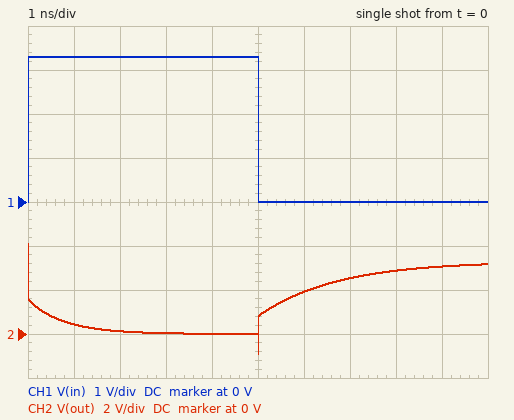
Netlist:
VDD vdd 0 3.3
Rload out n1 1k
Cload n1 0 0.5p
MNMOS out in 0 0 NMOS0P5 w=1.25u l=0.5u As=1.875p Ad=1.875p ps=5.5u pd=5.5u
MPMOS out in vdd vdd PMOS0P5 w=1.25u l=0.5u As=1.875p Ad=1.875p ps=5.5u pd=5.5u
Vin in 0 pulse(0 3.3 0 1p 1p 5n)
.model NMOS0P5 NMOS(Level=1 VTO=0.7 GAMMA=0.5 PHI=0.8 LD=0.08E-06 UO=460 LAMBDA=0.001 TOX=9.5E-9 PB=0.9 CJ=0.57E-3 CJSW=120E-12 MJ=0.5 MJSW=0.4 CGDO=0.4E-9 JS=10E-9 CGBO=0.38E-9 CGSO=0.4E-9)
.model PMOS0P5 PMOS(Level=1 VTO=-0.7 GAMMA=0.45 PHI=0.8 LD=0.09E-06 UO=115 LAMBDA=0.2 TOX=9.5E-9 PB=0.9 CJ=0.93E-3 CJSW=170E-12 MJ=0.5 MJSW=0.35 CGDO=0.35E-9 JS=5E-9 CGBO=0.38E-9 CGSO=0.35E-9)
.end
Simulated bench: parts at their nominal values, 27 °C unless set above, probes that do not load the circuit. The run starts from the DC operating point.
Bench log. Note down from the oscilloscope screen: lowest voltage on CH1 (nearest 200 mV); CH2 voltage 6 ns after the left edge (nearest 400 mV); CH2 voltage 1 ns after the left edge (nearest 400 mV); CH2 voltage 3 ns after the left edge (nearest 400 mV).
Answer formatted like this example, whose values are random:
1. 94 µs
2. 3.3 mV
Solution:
1. 0 V
2. 2.0 V
3. 400 mV
4. 0 V
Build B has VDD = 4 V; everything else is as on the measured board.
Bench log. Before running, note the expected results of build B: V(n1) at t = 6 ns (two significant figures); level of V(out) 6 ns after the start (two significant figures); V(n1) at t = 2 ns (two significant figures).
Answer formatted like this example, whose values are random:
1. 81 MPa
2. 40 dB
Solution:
1. 2.0 V
2. 2.7 V
3. 400 mV
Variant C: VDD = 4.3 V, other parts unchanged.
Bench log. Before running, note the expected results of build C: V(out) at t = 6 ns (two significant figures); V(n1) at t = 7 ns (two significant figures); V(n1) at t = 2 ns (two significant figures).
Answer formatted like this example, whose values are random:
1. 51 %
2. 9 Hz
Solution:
1. 3.0 V
2. 3.3 V
3. 450 mV
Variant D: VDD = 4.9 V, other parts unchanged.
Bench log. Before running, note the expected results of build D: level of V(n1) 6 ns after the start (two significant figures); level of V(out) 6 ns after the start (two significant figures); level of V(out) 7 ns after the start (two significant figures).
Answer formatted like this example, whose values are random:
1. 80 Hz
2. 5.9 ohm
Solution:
1. 2.8 V
2. 3.7 V
3. 4.4 V
